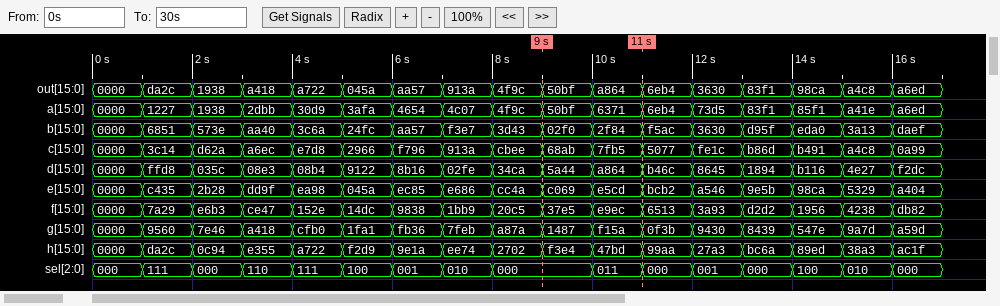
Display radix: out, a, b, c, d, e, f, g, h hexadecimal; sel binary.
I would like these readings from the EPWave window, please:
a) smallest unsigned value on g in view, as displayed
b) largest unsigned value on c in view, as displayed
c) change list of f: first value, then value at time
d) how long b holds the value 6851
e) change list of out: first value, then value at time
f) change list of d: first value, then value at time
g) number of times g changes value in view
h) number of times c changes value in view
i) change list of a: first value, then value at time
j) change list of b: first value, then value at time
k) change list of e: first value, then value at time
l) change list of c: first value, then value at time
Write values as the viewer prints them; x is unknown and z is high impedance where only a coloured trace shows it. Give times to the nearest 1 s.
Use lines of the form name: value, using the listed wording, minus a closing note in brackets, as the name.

smallest unsigned value on g in view, as displayed: 0000
largest unsigned value on c in view, as displayed: fe1c
change list of f: first value, then value at time: 0000, 7a29 at 1 s, e6b3 at 2 s, ce47 at 3 s, 152e at 4 s, 14dc at 5 s, 9838 at 6 s, 1bb9 at 7 s, 20c5 at 8 s, 37e5 at 9 s, e9ec at 10 s, 6513 at 11 s, 3a93 at 12 s, d2d2 at 13 s, 1956 at 14 s, 4238 at 15 s, db82 at 16 s
how long b holds the value 6851: 1 s
change list of out: first value, then value at time: 0000, da2c at 1 s, 1938 at 2 s, a418 at 3 s, a722 at 4 s, 045a at 5 s, aa57 at 6 s, 913a at 7 s, 4f9c at 8 s, 50bf at 9 s, a864 at 10 s, 6eb4 at 11 s, 3630 at 12 s, 83f1 at 13 s, 98ca at 14 s, a4c8 at 15 s, a6ed at 16 s
change list of d: first value, then value at time: 0000, ffd8 at 1 s, 035c at 2 s, 08e3 at 3 s, 08b4 at 4 s, 9122 at 5 s, 8b16 at 6 s, 02fe at 7 s, 34ca at 8 s, 5a44 at 9 s, a864 at 10 s, b46c at 11 s, 8645 at 12 s, 1894 at 13 s, b116 at 14 s, 4e27 at 15 s, f2dc at 16 s
number of times g changes value in view: 16
number of times c changes value in view: 16
change list of a: first value, then value at time: 0000, 1227 at 1 s, 1938 at 2 s, 2dbb at 3 s, 30d9 at 4 s, 3afa at 5 s, 4654 at 6 s, 4c07 at 7 s, 4f9c at 8 s, 50bf at 9 s, 6371 at 10 s, 6eb4 at 11 s, 73d5 at 12 s, 83f1 at 13 s, 85f1 at 14 s, a41e at 15 s, a6ed at 16 s
change list of b: first value, then value at time: 0000, 6851 at 1 s, 573e at 2 s, aa40 at 3 s, 3c6a at 4 s, 24fc at 5 s, aa57 at 6 s, f3e7 at 7 s, 3d43 at 8 s, 02f0 at 9 s, 2f84 at 10 s, f5ac at 11 s, 3630 at 12 s, d95f at 13 s, eda0 at 14 s, 3a13 at 15 s, daef at 16 s
change list of e: first value, then value at time: 0000, c435 at 1 s, 2b28 at 2 s, dd9f at 3 s, ea98 at 4 s, 045a at 5 s, ec85 at 6 s, e686 at 7 s, cc4a at 8 s, c069 at 9 s, e5cd at 10 s, bcb2 at 11 s, a546 at 12 s, 9e5b at 13 s, 98ca at 14 s, 5329 at 15 s, a404 at 16 s
change list of c: first value, then value at time: 0000, 3c14 at 1 s, d62a at 2 s, a6ec at 3 s, e7d8 at 4 s, 2966 at 5 s, f796 at 6 s, 913a at 7 s, cbee at 8 s, 68ab at 9 s, 7fb5 at 10 s, 5077 at 11 s, fe1c at 12 s, b86d at 13 s, b491 at 14 s, a4c8 at 15 s, 0a99 at 16 s
